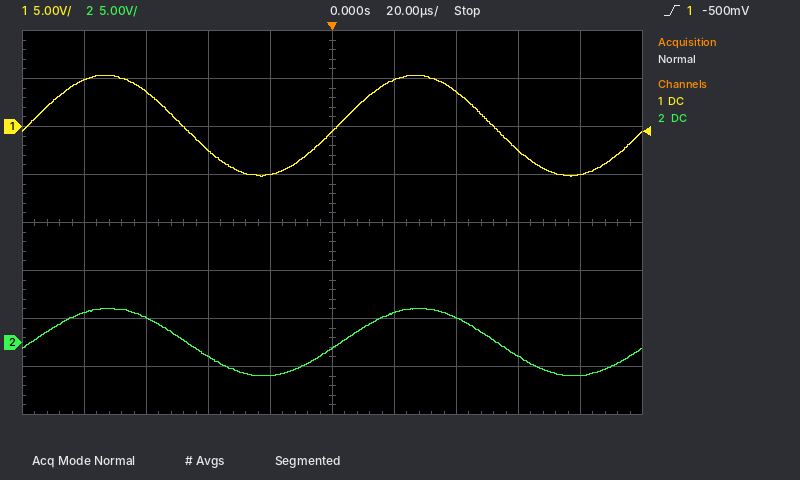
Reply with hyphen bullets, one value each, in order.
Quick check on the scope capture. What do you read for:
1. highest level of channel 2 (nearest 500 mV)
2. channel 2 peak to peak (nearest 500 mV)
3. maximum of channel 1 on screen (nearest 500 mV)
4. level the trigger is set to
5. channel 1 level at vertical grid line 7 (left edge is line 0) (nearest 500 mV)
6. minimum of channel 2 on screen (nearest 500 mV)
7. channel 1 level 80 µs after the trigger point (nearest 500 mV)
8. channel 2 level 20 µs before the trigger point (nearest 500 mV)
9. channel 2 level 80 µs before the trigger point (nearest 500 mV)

- 3.5 V
- 7.0 V
- 5.5 V
- -500 mV
- 3.5 V
- -3.5 V
- -5.0 V
- -3.5 V
- 3.0 V
